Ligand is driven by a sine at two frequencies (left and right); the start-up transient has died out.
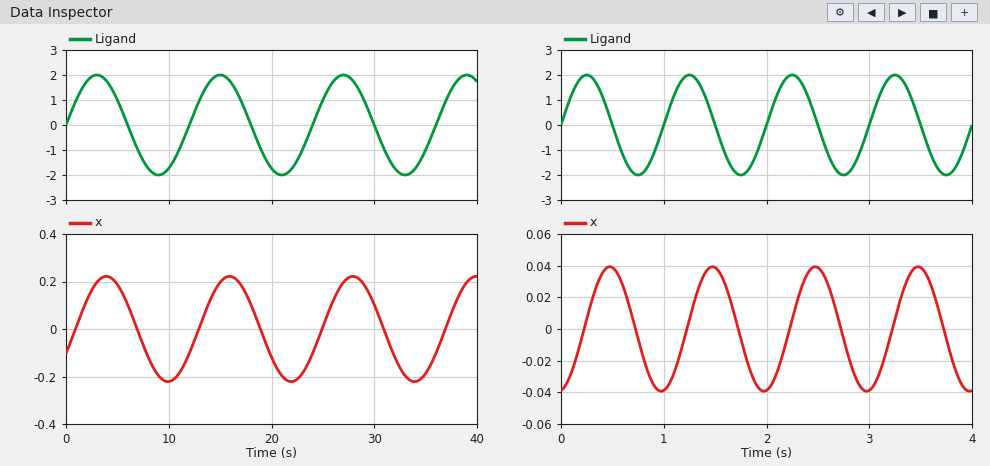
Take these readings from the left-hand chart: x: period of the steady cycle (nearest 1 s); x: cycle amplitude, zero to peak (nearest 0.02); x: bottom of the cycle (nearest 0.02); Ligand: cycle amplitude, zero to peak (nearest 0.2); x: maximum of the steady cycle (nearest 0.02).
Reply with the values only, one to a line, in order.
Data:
12 s
0.22
-0.22
2.0
0.22
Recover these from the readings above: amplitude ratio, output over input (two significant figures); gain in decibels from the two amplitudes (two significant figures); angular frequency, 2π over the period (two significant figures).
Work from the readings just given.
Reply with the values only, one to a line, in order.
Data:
0.11
-19 dB
0.52 rad/s
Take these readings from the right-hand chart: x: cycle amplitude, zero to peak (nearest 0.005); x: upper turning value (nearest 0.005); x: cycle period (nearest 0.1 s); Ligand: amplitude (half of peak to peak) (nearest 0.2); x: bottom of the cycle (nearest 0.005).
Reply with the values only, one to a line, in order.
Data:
0.040
0.040
1.0 s
2.0
-0.040
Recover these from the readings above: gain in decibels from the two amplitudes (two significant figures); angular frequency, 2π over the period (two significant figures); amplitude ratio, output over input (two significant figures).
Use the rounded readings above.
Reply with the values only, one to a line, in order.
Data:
-34 dB
6.3 rad/s
0.020
